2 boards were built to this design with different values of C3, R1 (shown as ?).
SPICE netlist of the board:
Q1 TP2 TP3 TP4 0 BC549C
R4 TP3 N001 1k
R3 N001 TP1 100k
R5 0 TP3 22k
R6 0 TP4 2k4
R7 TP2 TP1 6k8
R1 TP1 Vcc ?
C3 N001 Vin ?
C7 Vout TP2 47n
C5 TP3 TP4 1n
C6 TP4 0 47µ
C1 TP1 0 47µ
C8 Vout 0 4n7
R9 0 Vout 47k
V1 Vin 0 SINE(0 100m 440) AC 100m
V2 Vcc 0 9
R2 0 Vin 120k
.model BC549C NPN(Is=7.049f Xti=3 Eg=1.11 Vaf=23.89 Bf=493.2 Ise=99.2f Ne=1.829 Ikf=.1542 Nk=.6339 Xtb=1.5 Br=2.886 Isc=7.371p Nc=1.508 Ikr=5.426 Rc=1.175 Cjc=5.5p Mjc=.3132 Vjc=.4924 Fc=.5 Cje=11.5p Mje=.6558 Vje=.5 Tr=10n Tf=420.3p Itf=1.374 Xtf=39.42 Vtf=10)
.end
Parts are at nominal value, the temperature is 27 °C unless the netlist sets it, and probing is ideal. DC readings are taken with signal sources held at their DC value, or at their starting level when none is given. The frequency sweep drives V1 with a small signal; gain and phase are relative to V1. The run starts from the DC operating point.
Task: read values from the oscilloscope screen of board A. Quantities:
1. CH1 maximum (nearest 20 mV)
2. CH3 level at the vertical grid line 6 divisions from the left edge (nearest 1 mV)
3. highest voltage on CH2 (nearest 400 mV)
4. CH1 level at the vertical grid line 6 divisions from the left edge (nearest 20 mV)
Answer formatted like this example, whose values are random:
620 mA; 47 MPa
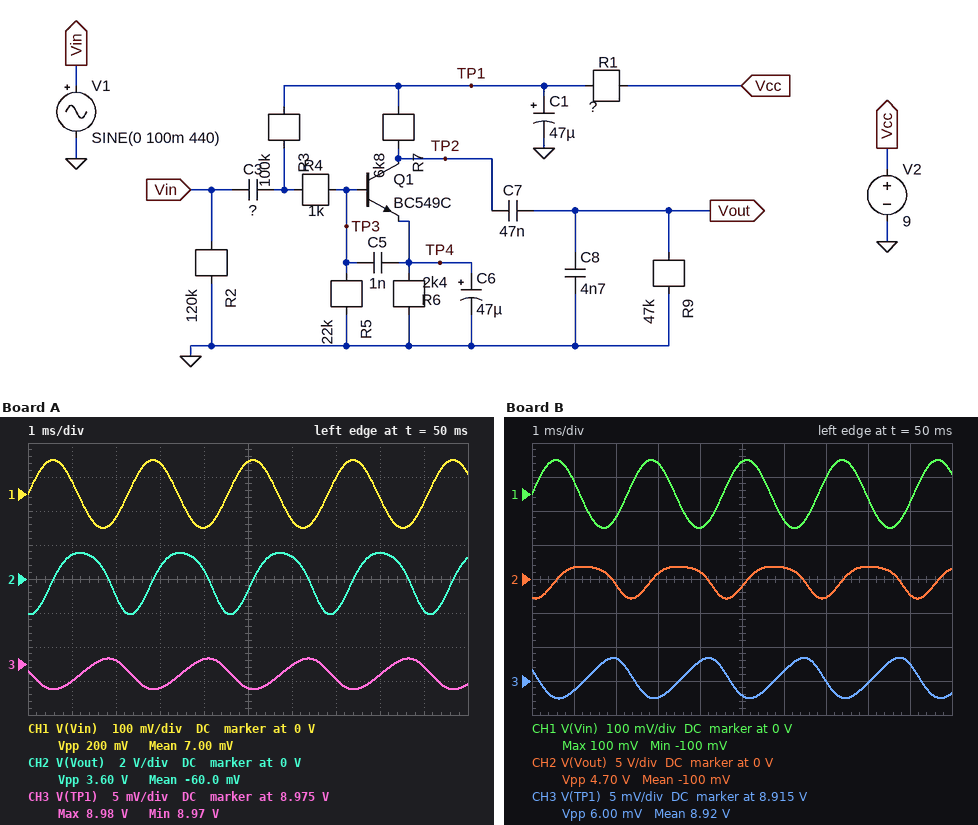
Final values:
100 mV; 8.975 V; 1.6 V; -80 mV
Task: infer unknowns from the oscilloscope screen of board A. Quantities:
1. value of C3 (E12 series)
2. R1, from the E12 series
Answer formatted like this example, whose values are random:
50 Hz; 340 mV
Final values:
8.2 nF; 56 Ω
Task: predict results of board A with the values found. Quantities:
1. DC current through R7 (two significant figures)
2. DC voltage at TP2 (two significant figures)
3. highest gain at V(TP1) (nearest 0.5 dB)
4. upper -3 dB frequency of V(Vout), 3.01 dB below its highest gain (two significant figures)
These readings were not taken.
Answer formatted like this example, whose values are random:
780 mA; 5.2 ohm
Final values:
400 µA; 6.3 V; -32.0 dB; 9.1 kHz
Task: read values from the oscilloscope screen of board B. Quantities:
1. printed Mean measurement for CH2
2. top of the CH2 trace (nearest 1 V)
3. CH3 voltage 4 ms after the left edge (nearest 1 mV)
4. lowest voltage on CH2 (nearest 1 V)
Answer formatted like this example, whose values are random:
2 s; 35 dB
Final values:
-100 mV; 2 V; 8.918 V; -3 V
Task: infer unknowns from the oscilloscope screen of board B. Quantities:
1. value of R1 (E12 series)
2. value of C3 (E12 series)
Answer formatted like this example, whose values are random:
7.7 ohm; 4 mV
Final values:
180 Ω; 12 nF
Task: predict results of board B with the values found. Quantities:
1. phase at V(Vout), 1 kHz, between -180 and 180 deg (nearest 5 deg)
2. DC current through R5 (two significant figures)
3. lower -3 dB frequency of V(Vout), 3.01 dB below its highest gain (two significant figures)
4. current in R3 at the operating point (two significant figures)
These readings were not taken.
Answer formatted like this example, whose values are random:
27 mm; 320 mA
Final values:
-140 deg; 72 µA; 760 Hz; 73 µA
